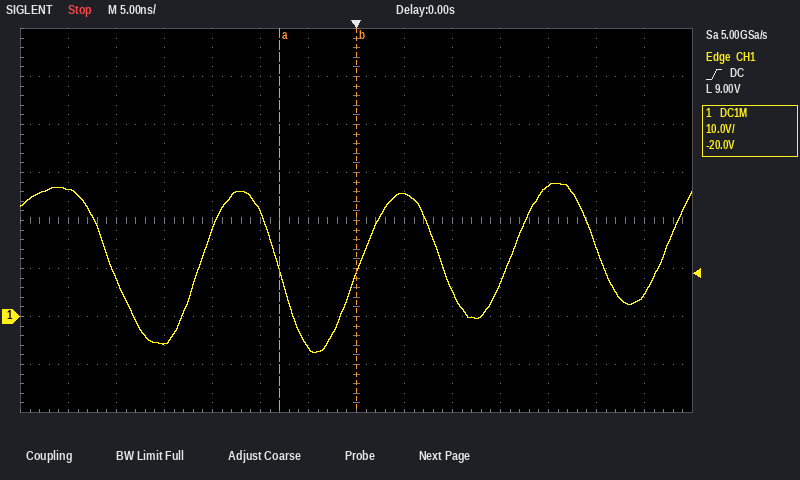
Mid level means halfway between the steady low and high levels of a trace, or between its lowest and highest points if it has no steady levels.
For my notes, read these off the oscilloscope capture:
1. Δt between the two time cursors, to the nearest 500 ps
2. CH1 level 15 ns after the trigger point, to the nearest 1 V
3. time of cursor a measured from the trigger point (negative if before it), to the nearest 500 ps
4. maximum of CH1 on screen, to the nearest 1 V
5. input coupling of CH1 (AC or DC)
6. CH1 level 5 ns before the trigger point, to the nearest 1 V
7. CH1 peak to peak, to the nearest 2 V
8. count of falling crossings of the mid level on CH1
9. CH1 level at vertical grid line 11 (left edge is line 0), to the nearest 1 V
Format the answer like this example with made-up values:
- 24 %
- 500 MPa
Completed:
- 8.0 ns
- 7 V
- -8.0 ns
- 28 V
- DC
- -6 V
- 36 V
- 4
- 27 V
